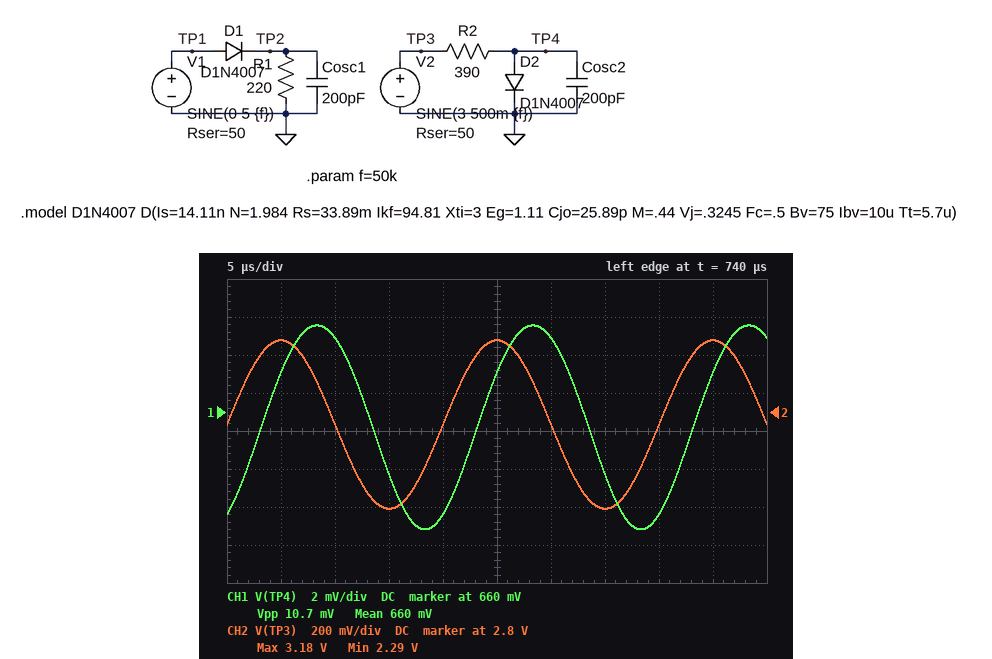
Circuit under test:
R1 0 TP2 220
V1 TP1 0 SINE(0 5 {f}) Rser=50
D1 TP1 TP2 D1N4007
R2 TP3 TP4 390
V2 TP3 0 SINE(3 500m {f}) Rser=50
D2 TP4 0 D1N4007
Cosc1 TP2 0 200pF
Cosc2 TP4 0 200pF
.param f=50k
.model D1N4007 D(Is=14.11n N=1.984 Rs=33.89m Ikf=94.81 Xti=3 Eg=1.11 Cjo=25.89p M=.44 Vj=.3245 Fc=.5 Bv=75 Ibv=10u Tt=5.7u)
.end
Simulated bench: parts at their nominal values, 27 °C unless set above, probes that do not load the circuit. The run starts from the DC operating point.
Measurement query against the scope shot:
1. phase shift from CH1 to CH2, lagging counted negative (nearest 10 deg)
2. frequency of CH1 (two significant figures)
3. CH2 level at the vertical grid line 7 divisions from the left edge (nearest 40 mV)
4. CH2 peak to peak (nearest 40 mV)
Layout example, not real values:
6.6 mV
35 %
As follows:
60 deg
50 kHz
2.28 V
880 mV
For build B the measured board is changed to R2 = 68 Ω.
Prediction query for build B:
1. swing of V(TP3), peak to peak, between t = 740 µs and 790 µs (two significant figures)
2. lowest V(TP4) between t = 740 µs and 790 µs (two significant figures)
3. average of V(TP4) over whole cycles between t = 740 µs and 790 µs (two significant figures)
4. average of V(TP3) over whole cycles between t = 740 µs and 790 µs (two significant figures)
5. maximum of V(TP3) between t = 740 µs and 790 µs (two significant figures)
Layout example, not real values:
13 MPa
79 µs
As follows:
580 mV
720 mV
730 mV
2.0 V
2.3 V
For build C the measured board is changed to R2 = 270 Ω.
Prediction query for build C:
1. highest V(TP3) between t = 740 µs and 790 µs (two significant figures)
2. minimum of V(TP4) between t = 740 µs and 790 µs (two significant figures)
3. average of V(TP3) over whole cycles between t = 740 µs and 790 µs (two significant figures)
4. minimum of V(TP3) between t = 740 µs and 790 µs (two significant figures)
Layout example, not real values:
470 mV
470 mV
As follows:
3.1 V
670 mV
2.6 V
2.2 V
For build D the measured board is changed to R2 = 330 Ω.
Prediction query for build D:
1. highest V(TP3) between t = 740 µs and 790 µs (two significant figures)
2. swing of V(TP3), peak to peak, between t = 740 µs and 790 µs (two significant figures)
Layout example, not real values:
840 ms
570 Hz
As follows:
3.1 V
870 mV
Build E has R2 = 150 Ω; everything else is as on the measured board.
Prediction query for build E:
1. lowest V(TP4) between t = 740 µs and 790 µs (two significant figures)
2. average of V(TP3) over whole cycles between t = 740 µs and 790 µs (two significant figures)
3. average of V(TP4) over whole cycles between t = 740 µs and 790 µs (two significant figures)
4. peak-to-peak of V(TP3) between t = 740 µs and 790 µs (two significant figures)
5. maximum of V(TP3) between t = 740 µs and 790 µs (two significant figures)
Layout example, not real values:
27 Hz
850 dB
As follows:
690 mV
2.4 V
700 mV
750 mV
2.8 V
